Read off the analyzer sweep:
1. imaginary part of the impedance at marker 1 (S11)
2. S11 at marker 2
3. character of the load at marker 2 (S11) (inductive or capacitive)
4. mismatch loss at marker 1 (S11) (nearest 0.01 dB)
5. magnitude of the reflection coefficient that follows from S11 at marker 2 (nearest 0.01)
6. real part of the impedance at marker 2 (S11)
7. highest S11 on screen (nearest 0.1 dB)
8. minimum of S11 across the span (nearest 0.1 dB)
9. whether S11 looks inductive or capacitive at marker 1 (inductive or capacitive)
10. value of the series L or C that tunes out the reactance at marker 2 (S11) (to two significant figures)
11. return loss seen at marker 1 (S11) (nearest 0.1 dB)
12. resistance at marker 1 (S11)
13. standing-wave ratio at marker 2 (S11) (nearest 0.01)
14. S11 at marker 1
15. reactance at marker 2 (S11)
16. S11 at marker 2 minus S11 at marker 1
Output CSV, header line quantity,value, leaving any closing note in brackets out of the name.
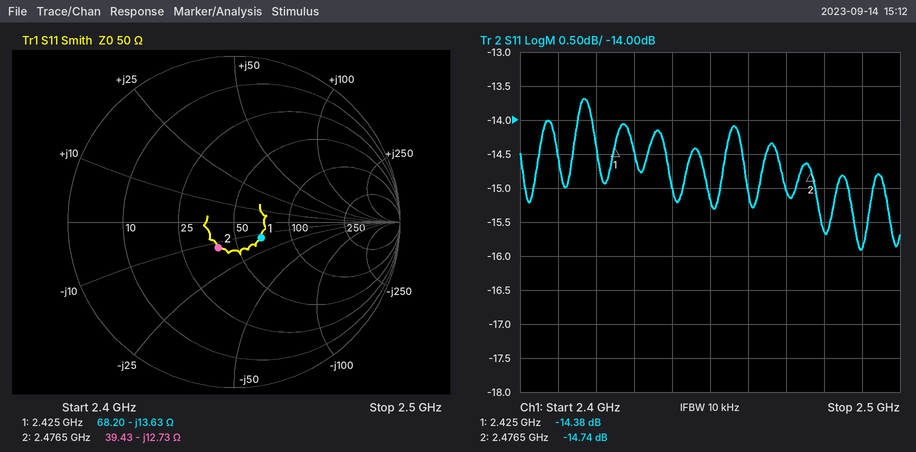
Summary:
quantity,value
imaginary part of the impedance at marker 1,-13.63 Ω
S11 at marker 2,-14.74 dB
character of the load at marker 2 (S11),capacitive
mismatch loss at marker 1 (S11),0.16 dB
magnitude of the reflection coefficient that follows from S11 at marker 2,0.18
real part of the impedance at marker 2,39.43 Ω
highest S11 on screen,-13.7 dB
minimum of S11 across the span,-15.9 dB
whether S11 looks inductive or capacitive at marker 1,capacitive
value of the series L or C that tunes out the reactance at marker 2 (S11),820 pH
return loss seen at marker 1 (S11),14.4 dB
resistance at marker 1,68.20 Ω
standing-wave ratio at marker 2 (S11),1.45
S11 at marker 1,-14.38 dB
reactance at marker 2,-12.73 Ω
S11 at marker 2 minus S11 at marker 1,-0.36 dB
